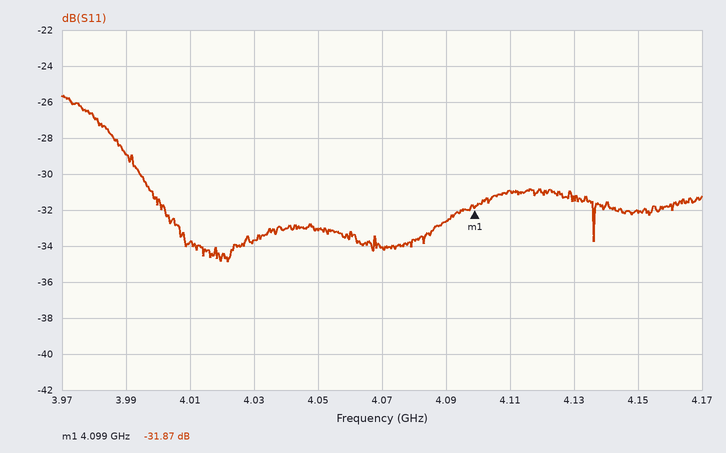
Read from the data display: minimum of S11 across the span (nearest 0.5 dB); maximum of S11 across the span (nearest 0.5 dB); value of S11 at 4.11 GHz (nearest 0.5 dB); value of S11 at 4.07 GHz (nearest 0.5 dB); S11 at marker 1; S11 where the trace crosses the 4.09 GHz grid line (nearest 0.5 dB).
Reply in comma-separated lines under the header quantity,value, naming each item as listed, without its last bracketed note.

quantity,value
minimum of S11 across the span,-35.0 dB
maximum of S11 across the span,-25.5 dB
value of S11 at 4.11 GHz,-31.0 dB
value of S11 at 4.07 GHz,-34.0 dB
S11 at marker 1,-31.87 dB
S11 where the trace crosses the 4.09 GHz grid line,-32.5 dB
